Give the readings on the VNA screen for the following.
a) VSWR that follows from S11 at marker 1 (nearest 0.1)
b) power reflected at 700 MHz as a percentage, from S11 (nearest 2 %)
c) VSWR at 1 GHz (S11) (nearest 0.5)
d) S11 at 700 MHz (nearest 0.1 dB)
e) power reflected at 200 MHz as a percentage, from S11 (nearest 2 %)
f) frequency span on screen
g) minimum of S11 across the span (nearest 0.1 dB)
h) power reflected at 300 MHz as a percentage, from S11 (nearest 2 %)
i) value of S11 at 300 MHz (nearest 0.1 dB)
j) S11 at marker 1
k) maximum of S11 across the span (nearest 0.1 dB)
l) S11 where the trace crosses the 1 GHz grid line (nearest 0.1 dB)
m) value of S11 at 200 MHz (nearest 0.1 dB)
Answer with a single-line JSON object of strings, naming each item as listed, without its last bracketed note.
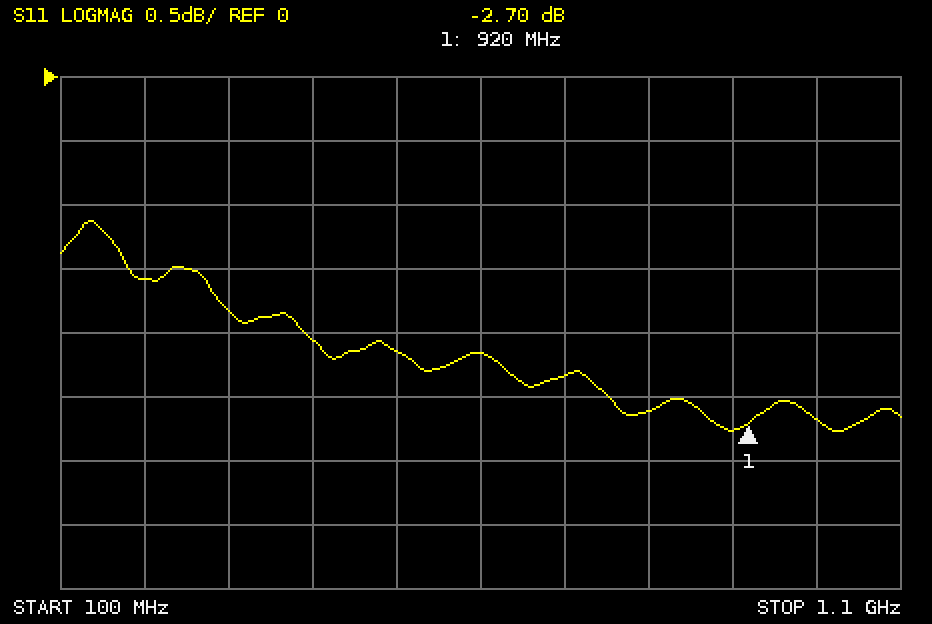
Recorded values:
{"VSWR that follows from S11 at marker 1": "6.5", "power reflected at 700 MHz as a percentage, from S11": "58 %", "VSWR at 1 GHz (S11)": "6.5", "S11 at 700 MHz": "-2.3 dB", "power reflected at 200 MHz as a percentage, from S11": "70 %", "frequency span on screen": "1 GHz", "minimum of S11 across the span": "-2.8 dB", "power reflected at 300 MHz as a percentage, from S11": "66 %", "value of S11 at 300 MHz": "-1.8 dB", "S11 at marker 1": "-2.70 dB", "maximum of S11 across the span": "-1.1 dB", "S11 where the trace crosses the 1 GHz grid line": "-2.7 dB", "value of S11 at 200 MHz": "-1.6 dB"}
